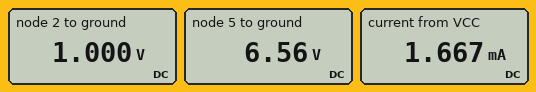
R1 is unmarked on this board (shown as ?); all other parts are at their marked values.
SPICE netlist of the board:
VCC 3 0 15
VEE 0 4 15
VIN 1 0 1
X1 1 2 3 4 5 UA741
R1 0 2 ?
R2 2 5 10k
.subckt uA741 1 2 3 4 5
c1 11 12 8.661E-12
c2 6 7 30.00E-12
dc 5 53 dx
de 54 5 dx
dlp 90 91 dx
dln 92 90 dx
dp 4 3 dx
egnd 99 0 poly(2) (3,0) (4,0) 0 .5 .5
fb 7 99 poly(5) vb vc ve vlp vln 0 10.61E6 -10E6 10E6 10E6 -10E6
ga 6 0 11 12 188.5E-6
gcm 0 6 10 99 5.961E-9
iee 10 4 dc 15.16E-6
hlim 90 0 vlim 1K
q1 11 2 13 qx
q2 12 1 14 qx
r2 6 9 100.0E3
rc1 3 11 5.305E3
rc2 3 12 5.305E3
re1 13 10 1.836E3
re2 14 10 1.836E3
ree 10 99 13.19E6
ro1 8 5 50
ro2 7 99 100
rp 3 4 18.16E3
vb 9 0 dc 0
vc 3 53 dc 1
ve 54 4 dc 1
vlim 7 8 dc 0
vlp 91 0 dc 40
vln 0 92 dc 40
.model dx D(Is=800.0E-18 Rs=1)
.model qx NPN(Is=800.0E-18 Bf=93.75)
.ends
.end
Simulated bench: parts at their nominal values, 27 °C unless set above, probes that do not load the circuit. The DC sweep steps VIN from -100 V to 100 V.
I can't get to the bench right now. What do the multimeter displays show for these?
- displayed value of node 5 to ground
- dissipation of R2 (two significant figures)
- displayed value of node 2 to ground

6.56 V
3.1 mW
1.000 V
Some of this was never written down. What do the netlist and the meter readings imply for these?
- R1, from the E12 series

1.8 kΩ
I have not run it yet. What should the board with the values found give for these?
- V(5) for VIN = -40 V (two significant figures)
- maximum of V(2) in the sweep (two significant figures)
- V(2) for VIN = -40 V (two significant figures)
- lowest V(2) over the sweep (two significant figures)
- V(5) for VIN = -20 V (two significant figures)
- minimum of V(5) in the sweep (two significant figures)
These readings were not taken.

-15 V
2.2 V
-2.2 V
-2.3 V
-15 V
-15 V
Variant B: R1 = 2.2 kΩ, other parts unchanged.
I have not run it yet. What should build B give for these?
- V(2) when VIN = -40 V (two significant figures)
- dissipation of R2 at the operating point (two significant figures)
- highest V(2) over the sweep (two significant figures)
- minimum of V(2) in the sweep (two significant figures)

-2.6 V
2.1 mW
2.6 V
-2.7 V
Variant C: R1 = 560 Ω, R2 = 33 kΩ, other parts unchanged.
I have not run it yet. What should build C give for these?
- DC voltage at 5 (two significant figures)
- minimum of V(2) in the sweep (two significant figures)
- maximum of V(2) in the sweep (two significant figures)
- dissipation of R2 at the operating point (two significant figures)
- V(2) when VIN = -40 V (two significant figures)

15 V
-250 mV
240 mV
6.3 mW
-240 mV
